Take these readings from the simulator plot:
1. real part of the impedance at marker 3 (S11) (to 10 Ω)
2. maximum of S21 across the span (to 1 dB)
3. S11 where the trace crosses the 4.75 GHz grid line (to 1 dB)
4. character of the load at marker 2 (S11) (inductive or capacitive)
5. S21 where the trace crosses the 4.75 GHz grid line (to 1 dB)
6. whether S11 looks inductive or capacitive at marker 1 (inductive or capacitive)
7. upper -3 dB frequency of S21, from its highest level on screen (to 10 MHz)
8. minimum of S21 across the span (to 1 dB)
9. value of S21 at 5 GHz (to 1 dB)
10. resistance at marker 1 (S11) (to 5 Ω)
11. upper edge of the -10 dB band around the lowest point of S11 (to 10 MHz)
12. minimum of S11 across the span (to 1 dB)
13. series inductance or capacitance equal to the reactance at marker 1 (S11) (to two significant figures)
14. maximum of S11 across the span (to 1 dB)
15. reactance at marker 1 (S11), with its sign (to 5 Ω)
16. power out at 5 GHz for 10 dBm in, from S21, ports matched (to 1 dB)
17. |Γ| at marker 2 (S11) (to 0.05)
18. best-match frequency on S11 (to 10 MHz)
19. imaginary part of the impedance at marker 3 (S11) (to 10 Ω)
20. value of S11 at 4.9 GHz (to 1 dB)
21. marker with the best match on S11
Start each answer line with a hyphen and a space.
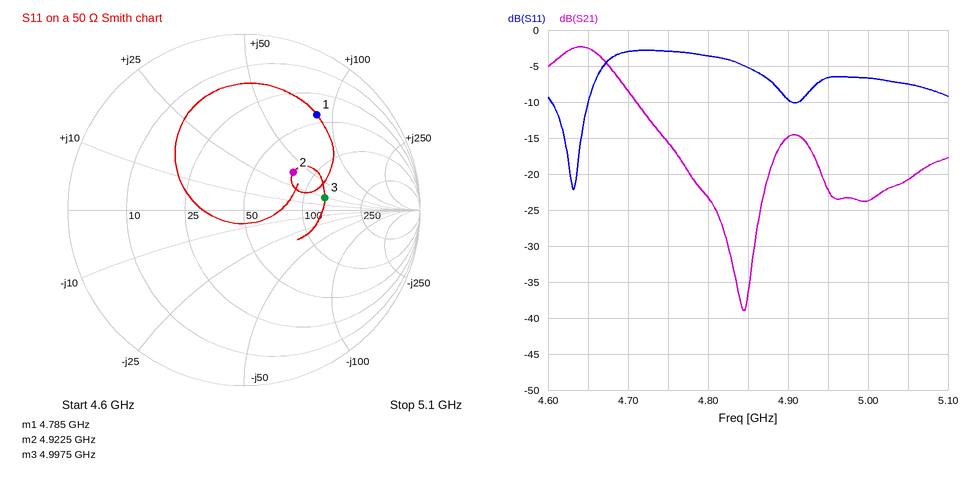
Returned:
- 130 Ω
- -2 dB
- -3 dB
- inductive
- -16 dB
- inductive
- 4.68 GHz
- -39 dB
- -24 dB
- 40 Ω
- 4.65 GHz
- -22 dB
- 2.8 nH
- -3 dB
- +85 Ω
- -14 dBm
- 0.35
- 4.63 GHz
- +20 Ω
- -10 dB
- marker 2
